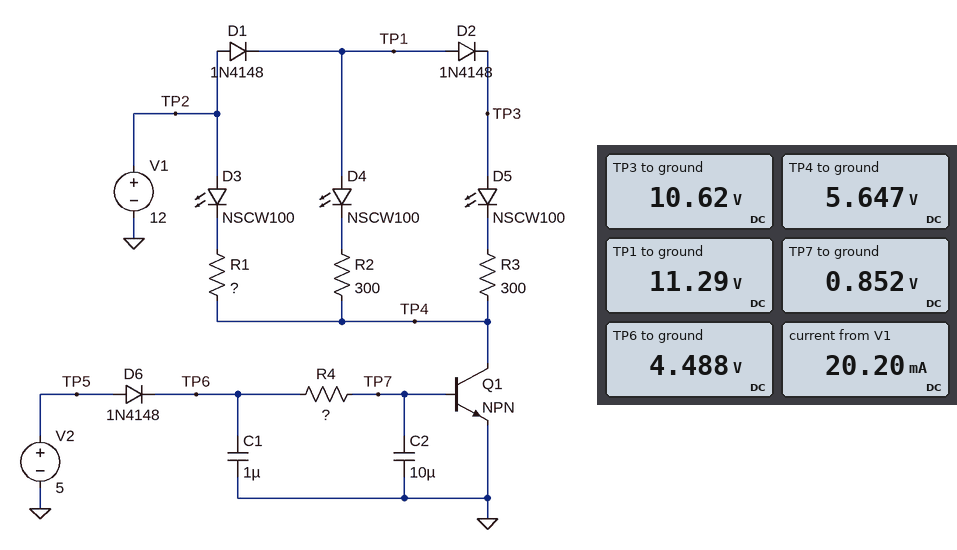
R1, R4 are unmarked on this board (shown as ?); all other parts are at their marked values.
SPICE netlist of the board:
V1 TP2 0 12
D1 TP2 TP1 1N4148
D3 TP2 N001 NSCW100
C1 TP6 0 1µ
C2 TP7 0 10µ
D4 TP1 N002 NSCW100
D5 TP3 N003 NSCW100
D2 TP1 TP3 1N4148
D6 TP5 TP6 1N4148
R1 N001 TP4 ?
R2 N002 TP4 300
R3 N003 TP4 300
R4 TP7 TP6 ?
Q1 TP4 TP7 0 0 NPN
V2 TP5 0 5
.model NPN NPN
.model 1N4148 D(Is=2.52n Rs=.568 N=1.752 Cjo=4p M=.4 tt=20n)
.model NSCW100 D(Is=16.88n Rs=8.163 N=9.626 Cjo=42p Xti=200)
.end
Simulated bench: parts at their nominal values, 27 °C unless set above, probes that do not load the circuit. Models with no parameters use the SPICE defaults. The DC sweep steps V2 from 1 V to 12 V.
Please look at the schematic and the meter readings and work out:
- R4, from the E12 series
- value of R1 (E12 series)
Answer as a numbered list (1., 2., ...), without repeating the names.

1. 18 kΩ
2. 470 Ω
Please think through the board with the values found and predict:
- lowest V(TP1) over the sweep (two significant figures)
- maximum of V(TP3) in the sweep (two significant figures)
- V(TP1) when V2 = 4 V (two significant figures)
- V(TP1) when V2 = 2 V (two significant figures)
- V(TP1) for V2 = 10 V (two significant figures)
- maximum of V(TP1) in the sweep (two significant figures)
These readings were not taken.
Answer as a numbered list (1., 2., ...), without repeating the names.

1. 11 V
2. 11 V
3. 11 V
4. 11 V
5. 11 V
6. 12 V
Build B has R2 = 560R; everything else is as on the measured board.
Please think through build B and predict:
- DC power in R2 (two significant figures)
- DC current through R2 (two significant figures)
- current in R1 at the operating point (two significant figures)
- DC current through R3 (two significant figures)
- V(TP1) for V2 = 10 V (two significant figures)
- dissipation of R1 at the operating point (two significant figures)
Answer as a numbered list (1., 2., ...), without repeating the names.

1. 16 mW
2. 5.3 mA
3. 7.6 mA
4. 7.3 mA
5. 11 V
6. 27 mW
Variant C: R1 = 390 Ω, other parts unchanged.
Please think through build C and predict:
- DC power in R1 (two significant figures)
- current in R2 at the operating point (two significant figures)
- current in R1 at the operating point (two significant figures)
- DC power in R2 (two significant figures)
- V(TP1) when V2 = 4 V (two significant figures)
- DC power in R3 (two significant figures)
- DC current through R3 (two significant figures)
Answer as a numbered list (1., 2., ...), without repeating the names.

1. 22 mW
2. 7.3 mA
3. 7.4 mA
4. 16 mW
5. 11 V
6. 8.8 mW
7. 5.4 mA
